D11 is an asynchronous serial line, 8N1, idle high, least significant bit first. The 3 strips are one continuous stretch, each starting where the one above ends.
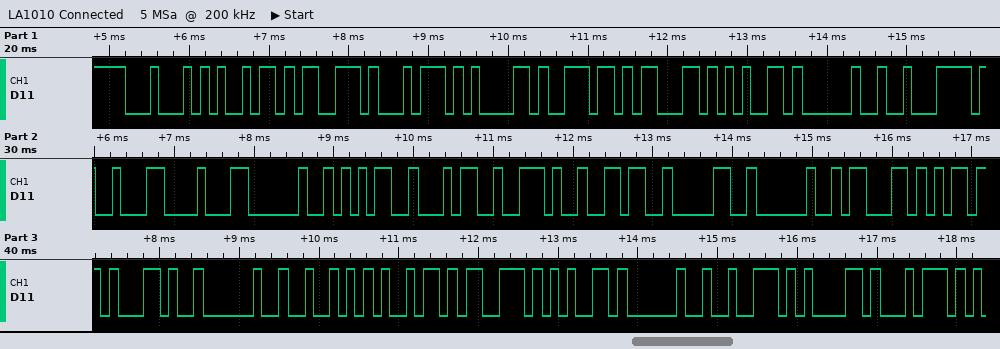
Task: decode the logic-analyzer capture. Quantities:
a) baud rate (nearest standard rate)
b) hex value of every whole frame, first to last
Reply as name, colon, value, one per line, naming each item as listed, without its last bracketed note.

baud rate: 9600 baud
hex value of every whole frame, first to last: 0x44 0x69 0x73 0x74 0x61 0x6E 0x63 0x65 0x20 0xE2 0x89 0x88 0x20 0x35 0x34 0x2E 0x36 0x30 0x20 0x63 0x6D 0x2C 0x20 0x52 0x69 0x73 0x65 0x20 0x72 0x61 0x74
